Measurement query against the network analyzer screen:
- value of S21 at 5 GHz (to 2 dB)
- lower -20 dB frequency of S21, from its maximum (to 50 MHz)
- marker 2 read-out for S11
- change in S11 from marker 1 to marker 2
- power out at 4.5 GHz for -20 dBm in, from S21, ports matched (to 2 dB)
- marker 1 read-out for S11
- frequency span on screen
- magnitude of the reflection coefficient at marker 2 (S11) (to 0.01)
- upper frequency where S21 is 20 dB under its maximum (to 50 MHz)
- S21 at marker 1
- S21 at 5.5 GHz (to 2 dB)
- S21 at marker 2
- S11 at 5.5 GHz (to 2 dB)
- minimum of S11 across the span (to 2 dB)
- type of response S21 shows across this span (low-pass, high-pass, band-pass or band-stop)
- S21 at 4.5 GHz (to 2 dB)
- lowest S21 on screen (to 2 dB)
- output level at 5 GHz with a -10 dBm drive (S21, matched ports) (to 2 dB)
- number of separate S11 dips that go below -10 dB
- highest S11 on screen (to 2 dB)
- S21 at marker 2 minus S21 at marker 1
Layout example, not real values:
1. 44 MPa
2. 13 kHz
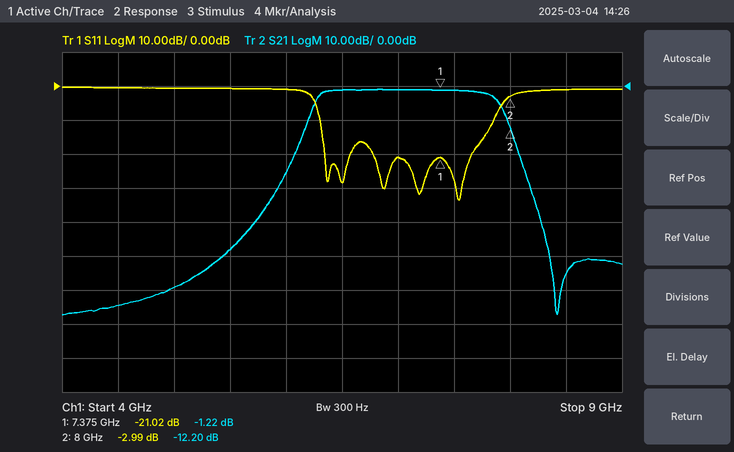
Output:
1. -60 dB
2. 6.05 GHz
3. -2.99 dB
4. 18.03 dB
5. -84 dBm
6. -21.02 dB
7. 5 GHz
8. 0.71
9. 8.10 GHz
10. -1.22 dB
11. -48 dB
12. -12.20 dB
13. 0 dB
14. -34 dB
15. band-pass
16. -64 dB
17. -68 dB
18. -70 dBm
19. 5
20. 0 dB
21. -10.98 dB
